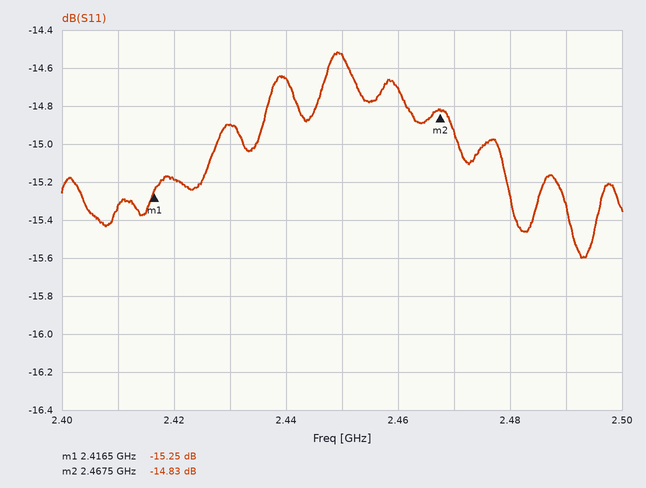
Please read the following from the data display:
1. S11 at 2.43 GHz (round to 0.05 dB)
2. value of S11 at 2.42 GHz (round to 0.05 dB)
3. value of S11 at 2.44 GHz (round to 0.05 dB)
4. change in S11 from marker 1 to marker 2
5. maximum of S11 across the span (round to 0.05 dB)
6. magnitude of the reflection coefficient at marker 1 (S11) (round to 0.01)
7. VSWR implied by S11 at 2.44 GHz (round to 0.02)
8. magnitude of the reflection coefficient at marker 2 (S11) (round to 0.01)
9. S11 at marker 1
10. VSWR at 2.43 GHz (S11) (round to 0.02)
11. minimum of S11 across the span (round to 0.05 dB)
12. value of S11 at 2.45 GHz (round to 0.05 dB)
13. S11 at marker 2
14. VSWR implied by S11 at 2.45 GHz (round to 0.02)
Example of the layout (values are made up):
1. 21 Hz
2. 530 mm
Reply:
1. -14.90 dB
2. -15.20 dB
3. -14.65 dB
4. 0.42 dB
5. -14.50 dB
6. 0.17
7. 1.46
8. 0.18
9. -15.25 dB
10. 1.44
11. -15.60 dB
12. -14.55 dB
13. -14.83 dB
14. 1.46
